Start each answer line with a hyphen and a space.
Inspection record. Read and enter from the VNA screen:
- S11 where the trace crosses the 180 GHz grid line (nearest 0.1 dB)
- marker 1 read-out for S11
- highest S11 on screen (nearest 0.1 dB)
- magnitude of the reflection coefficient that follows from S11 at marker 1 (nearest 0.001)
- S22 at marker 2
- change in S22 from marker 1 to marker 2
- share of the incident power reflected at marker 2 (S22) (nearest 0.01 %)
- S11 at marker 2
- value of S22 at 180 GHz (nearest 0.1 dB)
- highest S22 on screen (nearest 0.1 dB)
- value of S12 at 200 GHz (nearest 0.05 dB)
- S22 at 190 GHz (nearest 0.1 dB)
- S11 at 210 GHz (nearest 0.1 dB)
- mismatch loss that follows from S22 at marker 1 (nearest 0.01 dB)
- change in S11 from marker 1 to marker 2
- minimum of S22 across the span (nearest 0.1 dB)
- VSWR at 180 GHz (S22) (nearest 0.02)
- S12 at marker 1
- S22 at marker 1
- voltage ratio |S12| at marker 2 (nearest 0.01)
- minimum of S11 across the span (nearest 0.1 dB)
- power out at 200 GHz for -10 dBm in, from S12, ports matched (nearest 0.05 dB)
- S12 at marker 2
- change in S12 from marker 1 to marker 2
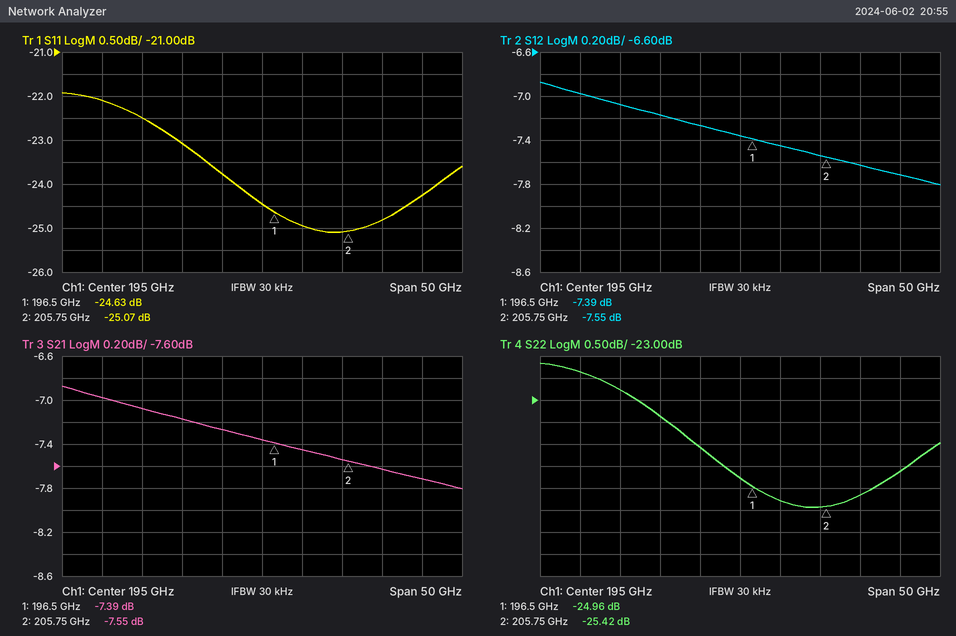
- -22.5 dB
- -24.63 dB
- -21.9 dB
- 0.059
- -25.42 dB
- -0.46 dB
- 0.29 %
- -25.07 dB
- -22.8 dB
- -22.2 dB
- -7.45 dB
- -24.1 dB
- -24.8 dB
- 0.01 dB
- -0.44 dB
- -25.4 dB
- 1.16
- -7.39 dB
- -24.96 dB
- 0.42
- -25.1 dB
- -17.45 dBm
- -7.55 dB
- -0.16 dB
